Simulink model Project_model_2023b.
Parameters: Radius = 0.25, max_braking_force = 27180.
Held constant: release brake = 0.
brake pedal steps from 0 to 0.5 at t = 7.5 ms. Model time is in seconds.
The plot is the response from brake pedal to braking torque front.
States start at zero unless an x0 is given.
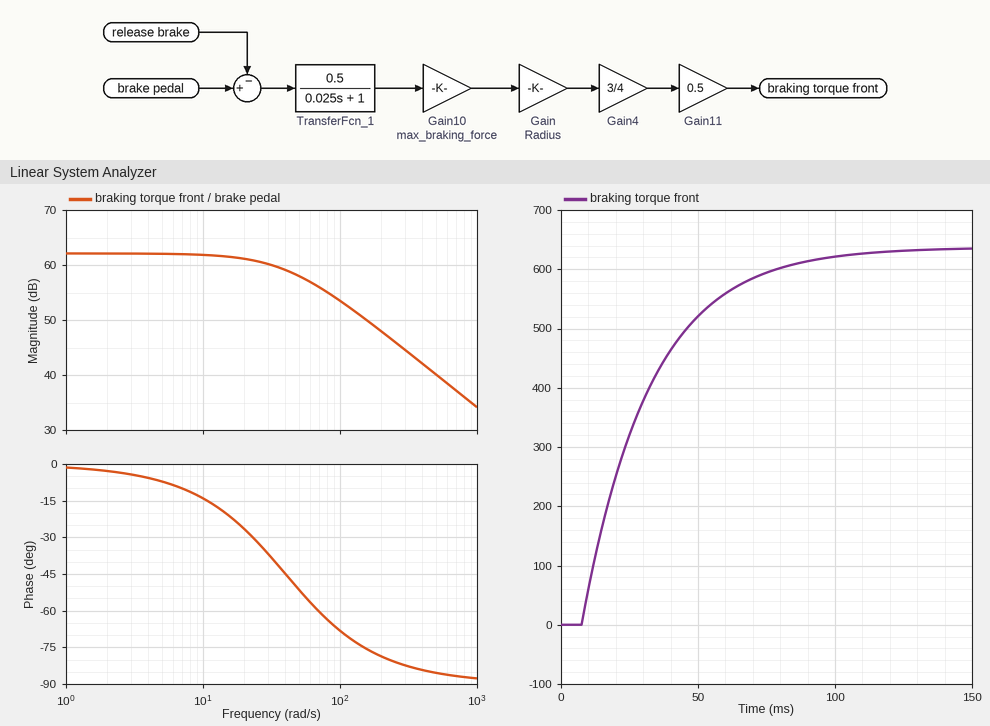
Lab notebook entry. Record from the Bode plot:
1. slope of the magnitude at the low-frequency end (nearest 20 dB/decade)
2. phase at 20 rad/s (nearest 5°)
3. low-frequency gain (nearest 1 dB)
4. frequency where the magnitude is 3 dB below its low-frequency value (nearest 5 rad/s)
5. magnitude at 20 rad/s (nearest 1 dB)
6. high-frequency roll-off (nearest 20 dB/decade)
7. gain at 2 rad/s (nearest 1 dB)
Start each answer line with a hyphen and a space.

- 0 dB/decade
- -25°
- 62 dB
- 40 rad/s
- 61 dB
- -20 dB/decade
- 62 dB
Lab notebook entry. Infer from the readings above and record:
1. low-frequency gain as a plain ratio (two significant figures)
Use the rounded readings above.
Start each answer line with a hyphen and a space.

- 1300
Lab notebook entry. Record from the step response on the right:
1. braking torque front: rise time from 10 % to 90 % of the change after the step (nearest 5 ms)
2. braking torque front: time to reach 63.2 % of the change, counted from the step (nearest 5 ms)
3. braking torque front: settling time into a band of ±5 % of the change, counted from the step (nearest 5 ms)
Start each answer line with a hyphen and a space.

- 55 ms
- 25 ms
- 75 ms
